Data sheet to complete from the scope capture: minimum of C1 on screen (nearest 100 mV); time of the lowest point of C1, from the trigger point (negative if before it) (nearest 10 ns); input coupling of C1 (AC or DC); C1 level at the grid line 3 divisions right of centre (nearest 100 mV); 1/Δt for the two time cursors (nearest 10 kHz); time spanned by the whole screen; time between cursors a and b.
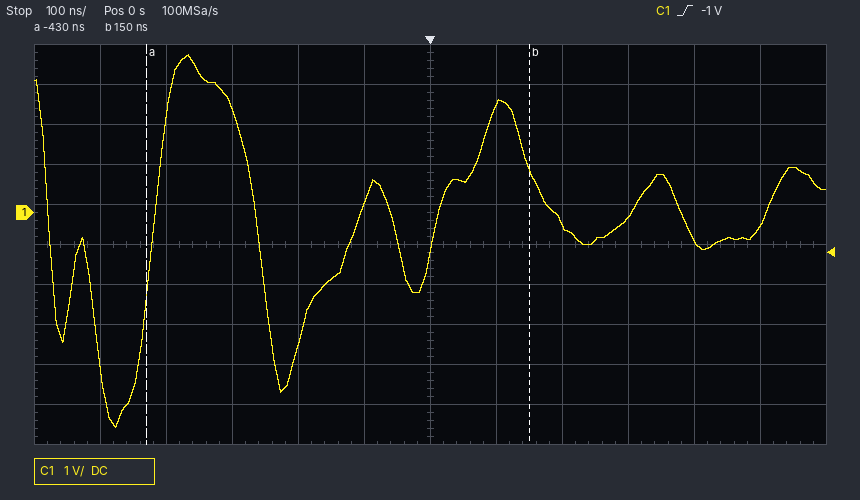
-5.4 V
-480 ns
DC
-100 mV
1.72 MHz
1.2 µs
580 ns
